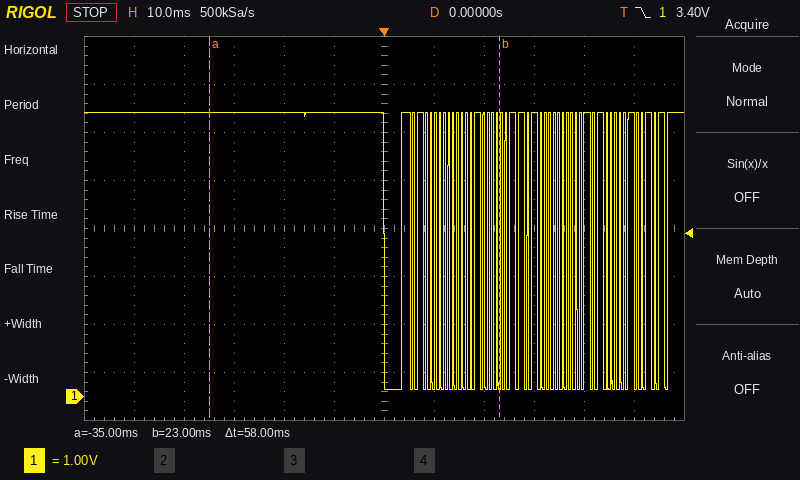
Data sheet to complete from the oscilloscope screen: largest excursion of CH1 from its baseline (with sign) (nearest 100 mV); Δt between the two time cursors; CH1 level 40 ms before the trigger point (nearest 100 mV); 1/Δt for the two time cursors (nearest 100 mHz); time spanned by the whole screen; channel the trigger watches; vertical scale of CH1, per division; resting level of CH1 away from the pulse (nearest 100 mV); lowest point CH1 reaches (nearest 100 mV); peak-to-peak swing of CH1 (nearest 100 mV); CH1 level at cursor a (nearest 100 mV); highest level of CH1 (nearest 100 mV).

-5.8 V
58 ms
5.9 V
17.2 Hz
120 ms
CH1
1 V
5.9 V
100 mV
5.8 V
5.9 V
5.9 V
